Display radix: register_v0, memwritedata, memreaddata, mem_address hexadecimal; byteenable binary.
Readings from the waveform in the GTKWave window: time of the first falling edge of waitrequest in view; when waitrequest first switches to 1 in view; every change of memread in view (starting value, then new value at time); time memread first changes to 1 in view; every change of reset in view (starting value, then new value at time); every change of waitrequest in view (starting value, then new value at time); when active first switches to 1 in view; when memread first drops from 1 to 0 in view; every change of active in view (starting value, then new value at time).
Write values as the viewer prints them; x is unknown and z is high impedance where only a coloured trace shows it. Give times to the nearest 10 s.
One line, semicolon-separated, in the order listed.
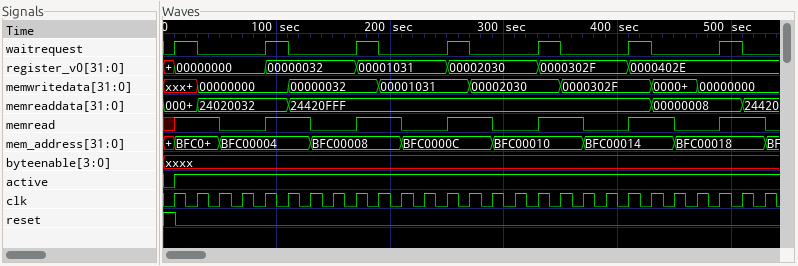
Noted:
30 s; 10 s; x, 1 at 10 s, 0 at 50 s, 1 at 90 s, 0 at 130 s, 1 at 170 s, 0 at 210 s, 1 at 250 s, 0 at 290 s, 1 at 330 s, 0 at 370 s, 1 at 410 s, 0 at 450 s, 1 at 490 s, 0 at 530 s; 10 s; 1, 0 at 10 s; 0, 1 at 10 s, 0 at 30 s, 1 at 90 s, 0 at 110 s, 1 at 170 s, 0 at 190 s, 1 at 250 s, 0 at 270 s, 1 at 330 s, 0 at 350 s, 1 at 410 s, 0 at 430 s, 1 at 490 s, 0 at 510 s; 10 s; 50 s; 0, 1 at 10 s
